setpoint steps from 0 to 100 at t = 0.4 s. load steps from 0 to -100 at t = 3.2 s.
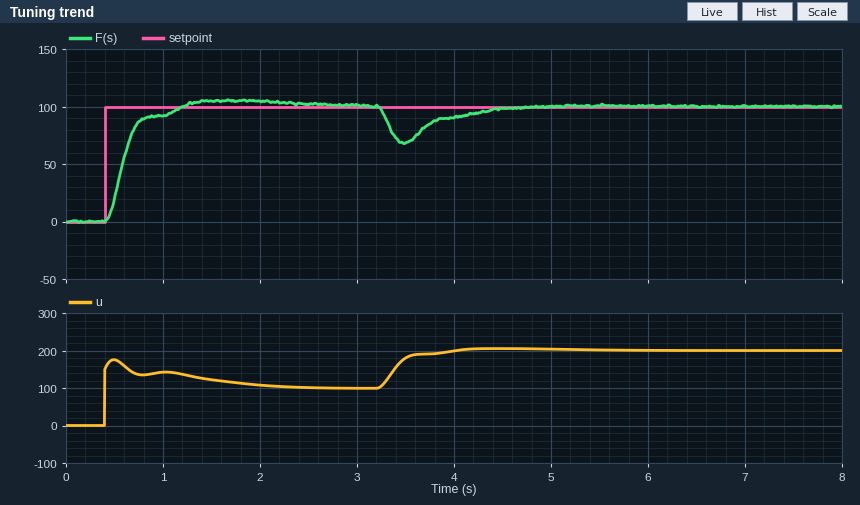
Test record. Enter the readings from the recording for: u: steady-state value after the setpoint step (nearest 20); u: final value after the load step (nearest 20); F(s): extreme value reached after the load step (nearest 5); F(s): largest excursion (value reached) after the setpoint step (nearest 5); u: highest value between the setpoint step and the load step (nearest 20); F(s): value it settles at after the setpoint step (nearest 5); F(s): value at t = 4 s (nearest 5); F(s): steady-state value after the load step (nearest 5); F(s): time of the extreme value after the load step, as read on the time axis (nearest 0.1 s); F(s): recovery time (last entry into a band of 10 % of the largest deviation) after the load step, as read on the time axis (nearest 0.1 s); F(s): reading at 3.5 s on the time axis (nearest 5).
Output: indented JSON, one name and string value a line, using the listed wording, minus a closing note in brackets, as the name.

{
  "u: steady-state value after the setpoint step": "100",
  "u: final value after the load step": "200",
  "F(s): extreme value reached after the load step": "70",
  "F(s): largest excursion (value reached) after the setpoint step": "105",
  "u: highest value between the setpoint step and the load step": "180",
  "F(s): value it settles at after the setpoint step": "100",
  "F(s): value at t = 4 s": "90",
  "F(s): steady-state value after the load step": "100",
  "F(s): time of the extreme value after the load step, as read on the time axis": "3.5 s",
  "F(s): recovery time (last entry into a band of 10 % of the largest deviation) after the load step, as read on the time axis": "4.4 s",
  "F(s): reading at 3.5 s on the time axis": "70"
}
